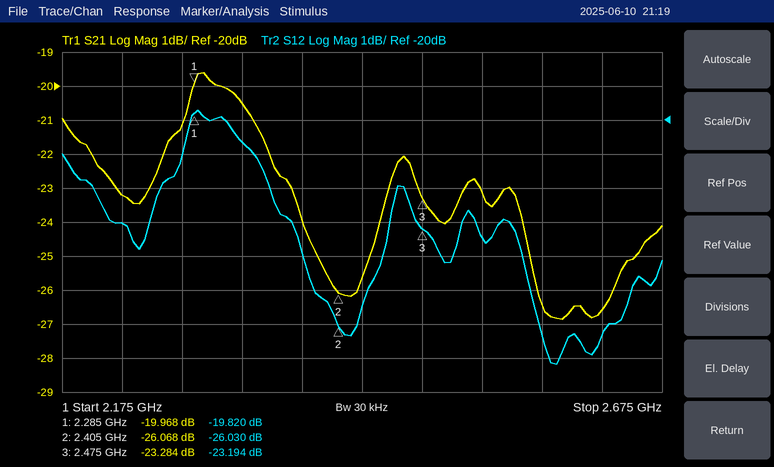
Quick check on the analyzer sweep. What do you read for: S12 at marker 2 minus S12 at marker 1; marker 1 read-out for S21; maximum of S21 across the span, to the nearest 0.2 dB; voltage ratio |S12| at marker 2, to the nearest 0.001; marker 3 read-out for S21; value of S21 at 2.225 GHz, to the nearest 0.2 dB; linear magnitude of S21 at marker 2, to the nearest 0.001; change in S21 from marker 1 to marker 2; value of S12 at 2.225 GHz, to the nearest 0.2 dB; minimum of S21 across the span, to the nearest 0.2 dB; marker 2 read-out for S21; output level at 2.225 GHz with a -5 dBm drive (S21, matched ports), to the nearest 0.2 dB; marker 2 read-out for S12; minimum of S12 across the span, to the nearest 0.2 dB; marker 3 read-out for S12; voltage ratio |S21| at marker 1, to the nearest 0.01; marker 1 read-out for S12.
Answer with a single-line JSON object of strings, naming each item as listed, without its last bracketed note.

{"S12 at marker 2 minus S12 at marker 1": "-6.210 dB", "marker 1 read-out for S21": "-19.968 dB", "maximum of S21 across the span, to the nearest 0.2 dB": "-19.6 dB", "voltage ratio |S12| at marker 2, to the nearest 0.001": "0.050", "marker 3 read-out for S21": "-23.284 dB", "value of S21 at 2.225 GHz, to the nearest 0.2 dB": "-23.2 dB", "linear magnitude of S21 at marker 2, to the nearest 0.001": "0.050", "change in S21 from marker 1 to marker 2": "-6.100 dB", "value of S12 at 2.225 GHz, to the nearest 0.2 dB": "-23.0 dB", "minimum of S21 across the span, to the nearest 0.2 dB": "-26.8 dB", "marker 2 read-out for S21": "-26.068 dB", "output level at 2.225 GHz with a -5 dBm drive (S21, matched ports), to the nearest 0.2 dB": "-28.2 dBm", "marker 2 read-out for S12": "-26.030 dB", "minimum of S12 across the span, to the nearest 0.2 dB": "-27.2 dB", "marker 3 read-out for S12": "-23.194 dB", "voltage ratio |S21| at marker 1, to the nearest 0.01": "0.10", "marker 1 read-out for S12": "-19.820 dB"}
